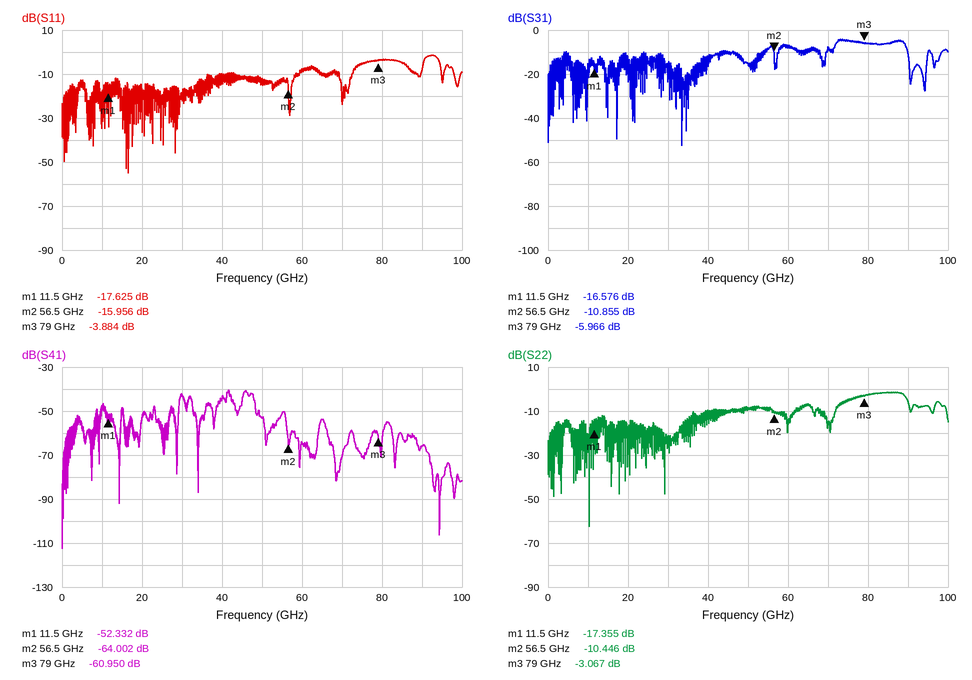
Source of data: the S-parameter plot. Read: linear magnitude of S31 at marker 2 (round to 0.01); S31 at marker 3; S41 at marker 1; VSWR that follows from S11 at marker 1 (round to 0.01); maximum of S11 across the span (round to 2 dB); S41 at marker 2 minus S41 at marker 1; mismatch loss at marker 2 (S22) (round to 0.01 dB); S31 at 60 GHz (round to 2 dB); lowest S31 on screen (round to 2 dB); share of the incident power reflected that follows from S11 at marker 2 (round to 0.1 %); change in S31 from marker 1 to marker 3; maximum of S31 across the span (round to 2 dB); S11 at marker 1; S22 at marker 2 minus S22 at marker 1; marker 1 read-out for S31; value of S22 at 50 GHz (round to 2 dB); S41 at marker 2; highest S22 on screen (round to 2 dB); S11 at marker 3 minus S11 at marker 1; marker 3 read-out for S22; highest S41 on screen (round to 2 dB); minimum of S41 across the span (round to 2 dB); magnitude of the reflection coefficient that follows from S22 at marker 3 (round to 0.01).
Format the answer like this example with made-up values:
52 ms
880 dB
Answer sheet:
0.29
-5.966 dB
-52.332 dB
1.30
-2 dB
-11.670 dB
0.41 dB
-8 dB
-52 dB
2.5 %
10.610 dB
-4 dB
-17.625 dB
6.909 dB
-16.576 dB
-8 dB
-64.002 dB
-2 dB
13.741 dB
-3.067 dB
-40 dB
-112 dB
0.70
